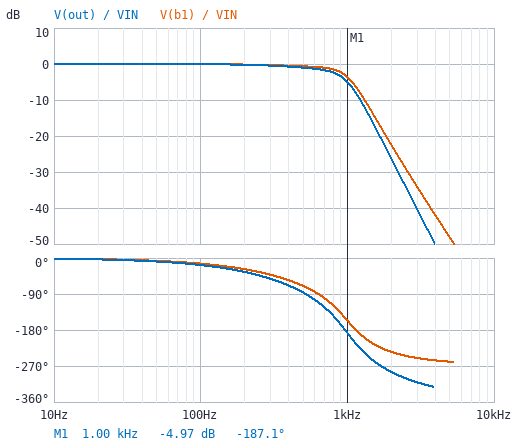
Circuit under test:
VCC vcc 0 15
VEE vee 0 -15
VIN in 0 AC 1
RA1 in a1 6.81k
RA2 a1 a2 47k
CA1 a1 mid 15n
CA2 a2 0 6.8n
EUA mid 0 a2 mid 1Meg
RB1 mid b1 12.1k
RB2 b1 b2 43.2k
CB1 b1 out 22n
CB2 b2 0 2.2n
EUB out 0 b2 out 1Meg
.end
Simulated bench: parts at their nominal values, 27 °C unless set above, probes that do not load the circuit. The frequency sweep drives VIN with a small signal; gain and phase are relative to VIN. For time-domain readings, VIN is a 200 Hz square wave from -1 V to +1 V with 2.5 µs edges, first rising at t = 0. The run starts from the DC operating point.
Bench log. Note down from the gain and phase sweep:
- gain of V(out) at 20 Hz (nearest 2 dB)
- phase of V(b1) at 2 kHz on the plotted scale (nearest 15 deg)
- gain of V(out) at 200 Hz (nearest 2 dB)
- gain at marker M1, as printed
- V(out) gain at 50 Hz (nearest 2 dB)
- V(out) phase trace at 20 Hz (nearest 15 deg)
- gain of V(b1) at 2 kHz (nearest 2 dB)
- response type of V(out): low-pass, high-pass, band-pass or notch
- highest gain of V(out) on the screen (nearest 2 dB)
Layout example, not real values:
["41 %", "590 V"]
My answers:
["0 dB", "-240 deg", "0 dB", "-4.97 dB", "0 dB", "0 deg", "-22 dB", "low-pass", "0 dB"]
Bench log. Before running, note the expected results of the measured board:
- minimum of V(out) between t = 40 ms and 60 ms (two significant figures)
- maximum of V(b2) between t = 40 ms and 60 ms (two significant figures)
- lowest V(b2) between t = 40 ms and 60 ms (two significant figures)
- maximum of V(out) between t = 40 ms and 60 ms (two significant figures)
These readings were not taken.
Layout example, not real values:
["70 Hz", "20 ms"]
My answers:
["-1.1 V", "1.1 V", "-1.1 V", "1.1 V"]
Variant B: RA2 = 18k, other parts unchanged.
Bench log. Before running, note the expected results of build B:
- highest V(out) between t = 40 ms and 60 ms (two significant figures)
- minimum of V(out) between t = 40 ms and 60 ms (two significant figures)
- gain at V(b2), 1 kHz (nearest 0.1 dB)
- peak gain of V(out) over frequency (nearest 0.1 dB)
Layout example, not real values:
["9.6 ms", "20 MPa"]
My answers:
["1.5 V", "-1.5 V", "0.9 dB", "2.2 dB"]
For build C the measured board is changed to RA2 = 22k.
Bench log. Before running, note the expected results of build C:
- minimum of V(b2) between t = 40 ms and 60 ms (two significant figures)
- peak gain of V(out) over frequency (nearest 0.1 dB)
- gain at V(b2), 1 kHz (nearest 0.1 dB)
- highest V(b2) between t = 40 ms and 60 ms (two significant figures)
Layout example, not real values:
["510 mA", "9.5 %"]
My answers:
["-1.4 V", "1.7 dB", "0.1 dB", "1.4 V"]
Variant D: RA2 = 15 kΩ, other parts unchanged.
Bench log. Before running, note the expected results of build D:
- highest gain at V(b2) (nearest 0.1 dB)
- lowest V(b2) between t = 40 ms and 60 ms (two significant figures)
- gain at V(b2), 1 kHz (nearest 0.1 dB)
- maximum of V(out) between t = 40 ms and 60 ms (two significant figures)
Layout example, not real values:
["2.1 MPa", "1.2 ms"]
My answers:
["2.6 dB", "-1.5 V", "1.5 dB", "1.5 V"]
